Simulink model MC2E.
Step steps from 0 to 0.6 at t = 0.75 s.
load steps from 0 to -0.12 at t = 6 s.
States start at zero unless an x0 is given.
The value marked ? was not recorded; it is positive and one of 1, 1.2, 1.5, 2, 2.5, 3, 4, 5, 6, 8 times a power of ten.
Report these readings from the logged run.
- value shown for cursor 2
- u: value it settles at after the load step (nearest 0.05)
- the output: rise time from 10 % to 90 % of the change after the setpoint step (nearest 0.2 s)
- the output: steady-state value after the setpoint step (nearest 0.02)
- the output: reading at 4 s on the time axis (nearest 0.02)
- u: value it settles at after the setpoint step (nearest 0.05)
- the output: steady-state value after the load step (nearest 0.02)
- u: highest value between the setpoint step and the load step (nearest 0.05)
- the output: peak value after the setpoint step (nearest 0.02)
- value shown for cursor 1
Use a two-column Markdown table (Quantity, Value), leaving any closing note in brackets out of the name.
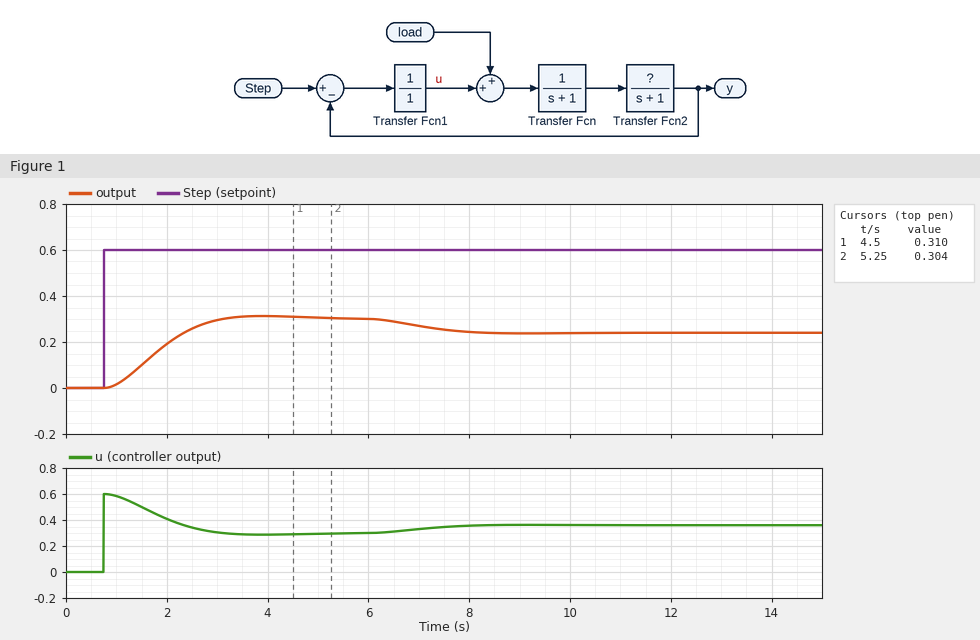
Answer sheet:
| Quantity | Value |
|---|---|
| value shown for cursor 2 | 0.304 |
| u: value it settles at after the load step | 0.35 |
| the output: rise time from 10 % to 90 % of the change after the setpoint step | 1.6 s |
| the output: steady-state value after the setpoint step | 0.30 |
| the output: reading at 4 s on the time axis | 0.32 |
| u: value it settles at after the setpoint step | 0.30 |
| the output: steady-state value after the load step | 0.24 |
| u: highest value between the setpoint step and the load step | 0.60 |
| the output: peak value after the setpoint step | 0.32 |
| value shown for cursor 1 | 0.310 |
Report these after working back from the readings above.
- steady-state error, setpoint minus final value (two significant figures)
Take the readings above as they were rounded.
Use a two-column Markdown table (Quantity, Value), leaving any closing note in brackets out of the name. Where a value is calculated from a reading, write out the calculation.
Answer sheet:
| Quantity | Value |
|---|---|
| steady-state error, setpoint minus final value | 0.6 - 0.3 = 0.30 |
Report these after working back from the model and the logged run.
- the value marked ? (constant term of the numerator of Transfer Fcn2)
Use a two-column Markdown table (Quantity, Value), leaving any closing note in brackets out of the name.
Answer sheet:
| Quantity | Value |
|---|---|
| the value marked ? | 1 |
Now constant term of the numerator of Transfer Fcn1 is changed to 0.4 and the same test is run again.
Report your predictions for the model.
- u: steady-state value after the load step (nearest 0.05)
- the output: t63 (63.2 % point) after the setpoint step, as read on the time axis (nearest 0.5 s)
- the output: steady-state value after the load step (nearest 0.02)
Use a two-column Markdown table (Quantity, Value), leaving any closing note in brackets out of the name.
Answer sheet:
| Quantity | Value |
|---|---|
| u: steady-state value after the load step | 0.20 |
| the output: t63 (63.2 % point) after the setpoint step, as read on the time axis | 2.5 s |
| the output: steady-state value after the load step | 0.08 |
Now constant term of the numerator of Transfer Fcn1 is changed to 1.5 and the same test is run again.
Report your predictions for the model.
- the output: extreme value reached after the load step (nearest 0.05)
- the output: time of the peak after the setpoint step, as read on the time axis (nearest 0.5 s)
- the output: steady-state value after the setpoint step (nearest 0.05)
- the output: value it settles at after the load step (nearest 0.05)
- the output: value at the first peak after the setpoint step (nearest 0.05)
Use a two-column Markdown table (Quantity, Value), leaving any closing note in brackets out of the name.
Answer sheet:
| Quantity | Value |
|---|---|
| the output: extreme value reached after the load step | 0.30 |
| the output: time of the peak after the setpoint step, as read on the time axis | 3.5 s |
| the output: steady-state value after the setpoint step | 0.35 |
| the output: value it settles at after the load step | 0.30 |
| the output: value at the first peak after the setpoint step | 0.40 |
